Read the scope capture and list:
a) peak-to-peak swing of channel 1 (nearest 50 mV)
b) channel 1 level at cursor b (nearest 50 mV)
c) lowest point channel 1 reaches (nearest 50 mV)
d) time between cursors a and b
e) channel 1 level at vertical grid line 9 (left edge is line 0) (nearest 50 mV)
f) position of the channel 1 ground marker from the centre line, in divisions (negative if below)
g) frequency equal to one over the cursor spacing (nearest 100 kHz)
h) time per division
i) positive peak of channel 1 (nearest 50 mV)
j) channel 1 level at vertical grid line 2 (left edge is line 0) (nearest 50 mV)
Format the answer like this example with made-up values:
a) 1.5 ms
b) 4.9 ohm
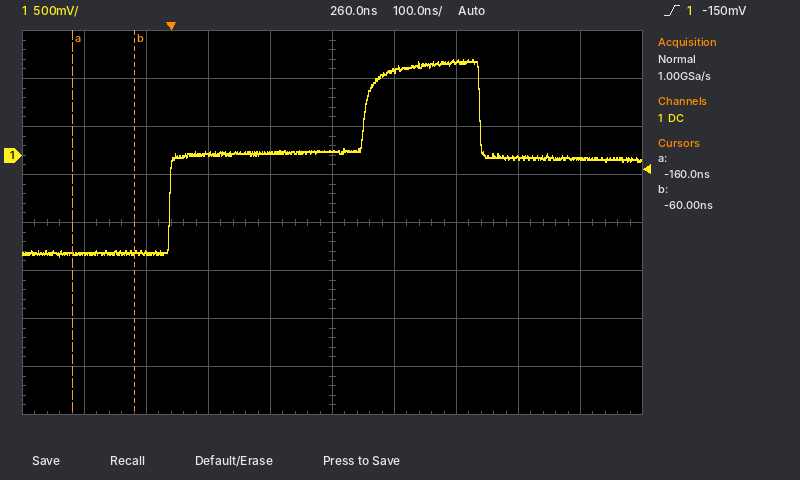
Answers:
a) 2.05 V
b) -1.00 V
c) -1.05 V
d) 100 ns
e) -50 mV
f) +1.4 div
g) 10.0 MHz
h) 100 ns
i) 1.00 V
j) -1.00 V
